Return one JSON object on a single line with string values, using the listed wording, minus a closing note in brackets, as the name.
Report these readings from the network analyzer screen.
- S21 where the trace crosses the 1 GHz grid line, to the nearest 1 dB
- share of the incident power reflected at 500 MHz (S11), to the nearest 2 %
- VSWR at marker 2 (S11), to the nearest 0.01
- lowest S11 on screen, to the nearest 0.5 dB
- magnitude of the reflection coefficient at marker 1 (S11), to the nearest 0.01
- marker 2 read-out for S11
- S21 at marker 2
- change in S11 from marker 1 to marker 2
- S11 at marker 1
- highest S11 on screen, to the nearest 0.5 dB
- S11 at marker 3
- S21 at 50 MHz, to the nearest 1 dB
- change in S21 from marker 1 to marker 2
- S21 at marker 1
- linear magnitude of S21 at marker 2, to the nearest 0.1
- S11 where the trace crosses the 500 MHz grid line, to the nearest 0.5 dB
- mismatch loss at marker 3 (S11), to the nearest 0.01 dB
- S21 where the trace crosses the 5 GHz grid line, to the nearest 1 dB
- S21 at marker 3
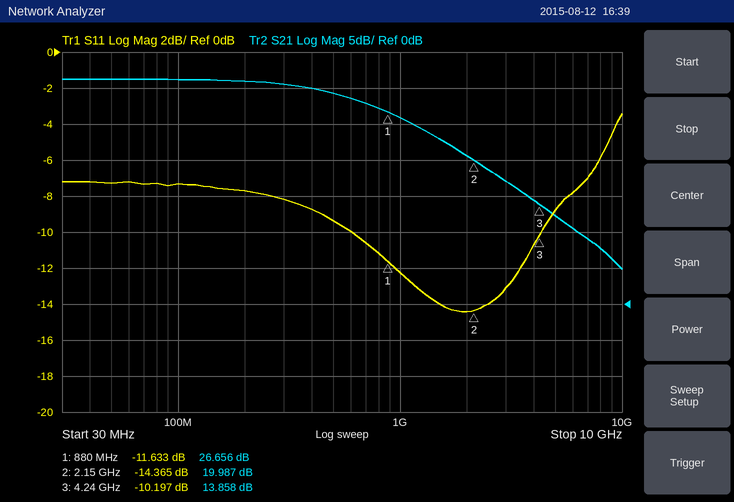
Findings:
{"S21 where the trace crosses the 1 GHz grid line, to the nearest 1 dB": "26 dB", "share of the incident power reflected at 500 MHz (S11), to the nearest 2 %": "12 %", "VSWR at marker 2 (S11), to the nearest 0.01": "1.47", "lowest S11 on screen, to the nearest 0.5 dB": "-14.5 dB", "magnitude of the reflection coefficient at marker 1 (S11), to the nearest 0.01": "0.26", "marker 2 read-out for S11": "-14.365 dB", "S21 at marker 2": "19.987 dB", "change in S11 from marker 1 to marker 2": "-2.732 dB", "S11 at marker 1": "-11.633 dB", "highest S11 on screen, to the nearest 0.5 dB": "-3.5 dB", "S11 at marker 3": "-10.197 dB", "S21 at 50 MHz, to the nearest 1 dB": "31 dB", "change in S21 from marker 1 to marker 2": "-6.669 dB", "S21 at marker 1": "26.656 dB", "linear magnitude of S21 at marker 2, to the nearest 0.1": "10.0", "S11 where the trace crosses the 500 MHz grid line, to the nearest 0.5 dB": "-9.5 dB", "mismatch loss at marker 3 (S11), to the nearest 0.01 dB": "0.44 dB", "S21 where the trace crosses the 5 GHz grid line, to the nearest 1 dB": "12 dB", "S21 at marker 3": "13.858 dB"}
